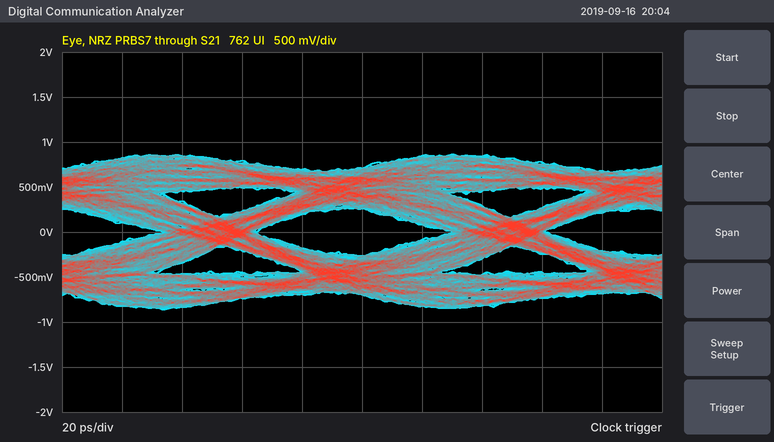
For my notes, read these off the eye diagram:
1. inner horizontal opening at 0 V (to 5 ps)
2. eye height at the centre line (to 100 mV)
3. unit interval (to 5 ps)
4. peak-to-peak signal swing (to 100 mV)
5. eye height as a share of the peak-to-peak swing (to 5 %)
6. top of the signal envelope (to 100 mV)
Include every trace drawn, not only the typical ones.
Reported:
65 ps
500 mV
95 ps
1.7 V
30 %
900 mV
